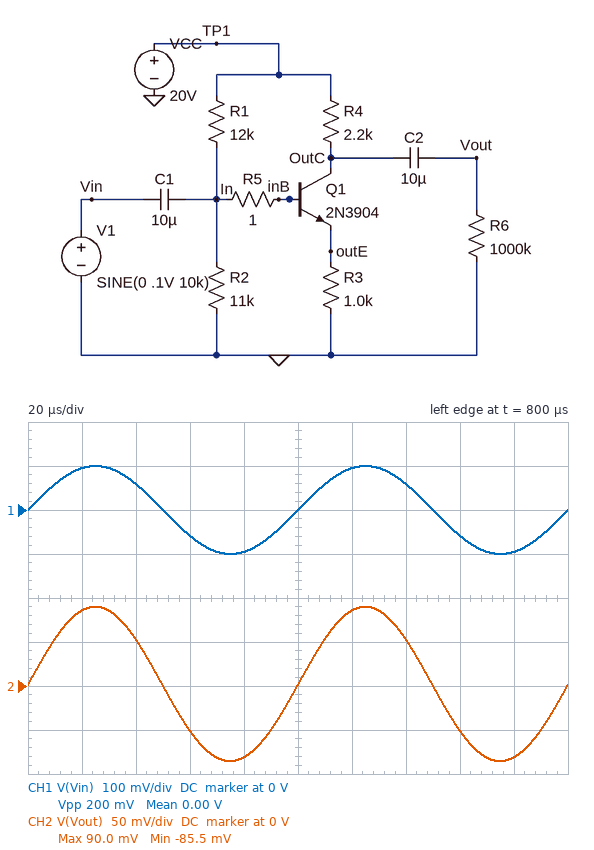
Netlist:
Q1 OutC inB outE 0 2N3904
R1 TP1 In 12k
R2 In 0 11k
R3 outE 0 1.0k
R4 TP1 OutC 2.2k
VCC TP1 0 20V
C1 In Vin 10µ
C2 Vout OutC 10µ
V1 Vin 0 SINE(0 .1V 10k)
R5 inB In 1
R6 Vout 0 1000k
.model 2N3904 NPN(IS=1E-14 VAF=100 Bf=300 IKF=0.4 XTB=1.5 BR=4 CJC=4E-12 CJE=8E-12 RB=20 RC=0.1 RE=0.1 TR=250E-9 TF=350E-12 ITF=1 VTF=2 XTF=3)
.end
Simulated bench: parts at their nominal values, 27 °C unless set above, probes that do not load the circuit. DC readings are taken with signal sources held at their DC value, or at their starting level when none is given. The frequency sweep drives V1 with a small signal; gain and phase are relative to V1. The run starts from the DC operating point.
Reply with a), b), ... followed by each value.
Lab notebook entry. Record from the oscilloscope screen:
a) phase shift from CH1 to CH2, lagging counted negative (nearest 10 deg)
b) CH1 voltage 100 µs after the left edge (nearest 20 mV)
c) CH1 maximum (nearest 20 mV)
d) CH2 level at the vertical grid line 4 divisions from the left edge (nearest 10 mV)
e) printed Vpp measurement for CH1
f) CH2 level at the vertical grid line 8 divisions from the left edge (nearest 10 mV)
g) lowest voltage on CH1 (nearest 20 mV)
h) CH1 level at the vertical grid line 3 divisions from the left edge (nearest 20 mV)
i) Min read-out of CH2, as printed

a) 0 deg
b) 0 V
c) 100 mV
d) -80 mV
e) 200 mV
f) -50 mV
g) -100 mV
h) -60 mV
i) -85.5 mV
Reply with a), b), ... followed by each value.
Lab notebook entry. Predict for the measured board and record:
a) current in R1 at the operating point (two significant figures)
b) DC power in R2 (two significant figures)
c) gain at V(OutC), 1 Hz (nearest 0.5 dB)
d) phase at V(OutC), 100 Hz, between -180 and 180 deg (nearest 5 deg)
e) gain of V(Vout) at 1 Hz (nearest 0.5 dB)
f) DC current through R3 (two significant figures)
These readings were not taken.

a) 1.1 mA
b) 4.8 mW
c) -29.0 dB
d) 15 deg
e) -29.0 dB
f) 6.5 mA
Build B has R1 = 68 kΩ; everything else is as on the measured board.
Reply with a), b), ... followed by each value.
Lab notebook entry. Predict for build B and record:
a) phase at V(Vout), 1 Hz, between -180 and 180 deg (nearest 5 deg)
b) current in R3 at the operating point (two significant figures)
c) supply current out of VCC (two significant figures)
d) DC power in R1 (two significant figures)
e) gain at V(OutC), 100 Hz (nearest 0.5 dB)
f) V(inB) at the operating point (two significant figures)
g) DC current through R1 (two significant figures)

a) -120 deg
b) 2.1 mA
c) 2.3 mA
d) 4.4 mW
e) 6.5 dB
f) 2.7 V
g) 250 µA
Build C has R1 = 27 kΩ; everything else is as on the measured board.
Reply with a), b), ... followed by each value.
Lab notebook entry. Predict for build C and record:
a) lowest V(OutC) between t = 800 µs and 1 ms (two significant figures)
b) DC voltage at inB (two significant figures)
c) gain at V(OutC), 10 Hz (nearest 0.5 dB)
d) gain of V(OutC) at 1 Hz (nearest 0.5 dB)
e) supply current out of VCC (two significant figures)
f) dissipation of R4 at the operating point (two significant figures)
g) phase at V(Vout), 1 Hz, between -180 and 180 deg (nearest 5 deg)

a) 8.9 V
b) 5.7 V
c) 6.5 dB
d) -0.5 dB
e) 5.5 mA
f) 54 mW
g) -115 deg
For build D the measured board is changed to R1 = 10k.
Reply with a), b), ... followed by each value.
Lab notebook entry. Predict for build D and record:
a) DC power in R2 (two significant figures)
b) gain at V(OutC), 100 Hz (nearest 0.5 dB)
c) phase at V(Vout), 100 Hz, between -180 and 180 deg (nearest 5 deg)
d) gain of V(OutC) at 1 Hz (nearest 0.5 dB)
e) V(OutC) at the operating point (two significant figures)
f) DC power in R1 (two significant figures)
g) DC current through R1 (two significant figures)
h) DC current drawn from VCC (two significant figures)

a) 4.9 mW
b) -1.0 dB
c) 15 deg
d) -28.5 dB
e) 6.7 V
f) 16 mW
g) 1.3 mA
h) 7.3 mA
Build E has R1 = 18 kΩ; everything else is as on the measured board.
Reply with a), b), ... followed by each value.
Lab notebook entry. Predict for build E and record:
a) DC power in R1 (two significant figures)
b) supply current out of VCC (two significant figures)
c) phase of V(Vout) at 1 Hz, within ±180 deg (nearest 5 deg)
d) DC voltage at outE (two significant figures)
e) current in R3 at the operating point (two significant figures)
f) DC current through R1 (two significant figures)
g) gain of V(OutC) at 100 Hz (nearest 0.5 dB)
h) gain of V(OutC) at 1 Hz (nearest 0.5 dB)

a) 9.4 mW
b) 6.9 mA
c) 90 deg
d) 6.3 V
e) 6.3 mA
f) 720 µA
g) -6.0 dB
h) -32.5 dB
